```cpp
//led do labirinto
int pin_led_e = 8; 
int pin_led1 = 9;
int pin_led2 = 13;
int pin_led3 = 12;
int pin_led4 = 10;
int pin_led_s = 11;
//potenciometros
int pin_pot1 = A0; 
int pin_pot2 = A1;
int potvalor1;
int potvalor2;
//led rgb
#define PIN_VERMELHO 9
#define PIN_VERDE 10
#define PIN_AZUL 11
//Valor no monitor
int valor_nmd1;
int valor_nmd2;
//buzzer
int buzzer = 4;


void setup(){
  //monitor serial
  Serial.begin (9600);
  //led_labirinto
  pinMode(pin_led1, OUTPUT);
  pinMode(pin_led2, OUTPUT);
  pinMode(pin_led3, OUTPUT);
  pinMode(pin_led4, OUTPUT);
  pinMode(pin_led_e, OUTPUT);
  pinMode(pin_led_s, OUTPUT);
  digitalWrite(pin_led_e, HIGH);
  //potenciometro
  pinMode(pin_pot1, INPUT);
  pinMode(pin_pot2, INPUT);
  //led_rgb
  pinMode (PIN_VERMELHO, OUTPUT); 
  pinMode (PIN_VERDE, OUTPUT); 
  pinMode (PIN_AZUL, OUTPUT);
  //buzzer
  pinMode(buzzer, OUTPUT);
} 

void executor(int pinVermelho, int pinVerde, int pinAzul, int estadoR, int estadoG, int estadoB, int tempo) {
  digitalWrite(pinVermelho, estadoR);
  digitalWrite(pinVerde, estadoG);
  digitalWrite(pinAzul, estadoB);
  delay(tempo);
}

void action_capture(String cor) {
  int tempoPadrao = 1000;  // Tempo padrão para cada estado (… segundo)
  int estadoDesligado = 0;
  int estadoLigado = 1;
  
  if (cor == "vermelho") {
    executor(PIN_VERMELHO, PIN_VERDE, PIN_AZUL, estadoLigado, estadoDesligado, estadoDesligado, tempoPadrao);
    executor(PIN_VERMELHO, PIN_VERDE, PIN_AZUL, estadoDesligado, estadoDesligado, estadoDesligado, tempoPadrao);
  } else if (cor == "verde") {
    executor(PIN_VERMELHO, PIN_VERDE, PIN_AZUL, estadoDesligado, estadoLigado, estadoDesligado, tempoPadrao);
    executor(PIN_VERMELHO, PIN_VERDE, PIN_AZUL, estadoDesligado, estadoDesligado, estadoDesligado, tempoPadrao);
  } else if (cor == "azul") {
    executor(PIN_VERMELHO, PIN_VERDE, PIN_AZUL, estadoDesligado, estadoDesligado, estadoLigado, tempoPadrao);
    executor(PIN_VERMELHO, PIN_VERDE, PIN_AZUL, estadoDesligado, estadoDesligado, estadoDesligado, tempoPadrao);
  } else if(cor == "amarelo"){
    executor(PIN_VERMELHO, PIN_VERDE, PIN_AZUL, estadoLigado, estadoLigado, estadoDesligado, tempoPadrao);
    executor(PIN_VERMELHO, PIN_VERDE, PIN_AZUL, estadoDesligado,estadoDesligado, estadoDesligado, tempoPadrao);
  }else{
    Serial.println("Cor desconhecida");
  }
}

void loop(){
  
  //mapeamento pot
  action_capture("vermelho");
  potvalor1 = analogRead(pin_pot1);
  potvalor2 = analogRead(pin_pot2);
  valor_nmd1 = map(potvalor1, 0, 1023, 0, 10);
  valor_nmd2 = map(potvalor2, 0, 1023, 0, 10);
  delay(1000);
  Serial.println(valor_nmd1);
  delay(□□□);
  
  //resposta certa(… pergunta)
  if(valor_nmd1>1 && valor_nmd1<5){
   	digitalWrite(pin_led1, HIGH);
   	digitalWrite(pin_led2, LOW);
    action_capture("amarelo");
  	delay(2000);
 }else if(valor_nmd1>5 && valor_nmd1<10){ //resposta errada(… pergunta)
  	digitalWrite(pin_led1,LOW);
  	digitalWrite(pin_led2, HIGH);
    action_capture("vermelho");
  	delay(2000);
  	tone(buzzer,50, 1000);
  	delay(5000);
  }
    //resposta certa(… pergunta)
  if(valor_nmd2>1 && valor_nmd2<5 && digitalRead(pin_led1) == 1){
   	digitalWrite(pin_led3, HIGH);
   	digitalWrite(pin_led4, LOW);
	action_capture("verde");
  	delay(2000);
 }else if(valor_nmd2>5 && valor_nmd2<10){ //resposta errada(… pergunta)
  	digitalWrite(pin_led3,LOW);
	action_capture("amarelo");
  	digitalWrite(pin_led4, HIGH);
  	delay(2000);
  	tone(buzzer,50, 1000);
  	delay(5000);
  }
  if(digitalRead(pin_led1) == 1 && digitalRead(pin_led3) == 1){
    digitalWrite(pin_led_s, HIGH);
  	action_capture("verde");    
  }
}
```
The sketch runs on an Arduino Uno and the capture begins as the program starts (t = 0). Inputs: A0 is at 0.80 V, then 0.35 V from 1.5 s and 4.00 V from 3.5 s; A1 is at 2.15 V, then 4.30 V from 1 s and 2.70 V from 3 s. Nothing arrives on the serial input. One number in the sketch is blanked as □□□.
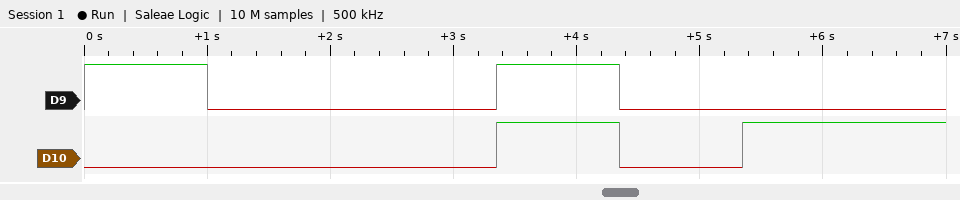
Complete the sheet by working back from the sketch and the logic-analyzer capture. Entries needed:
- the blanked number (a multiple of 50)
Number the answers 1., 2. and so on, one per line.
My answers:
1. 350
